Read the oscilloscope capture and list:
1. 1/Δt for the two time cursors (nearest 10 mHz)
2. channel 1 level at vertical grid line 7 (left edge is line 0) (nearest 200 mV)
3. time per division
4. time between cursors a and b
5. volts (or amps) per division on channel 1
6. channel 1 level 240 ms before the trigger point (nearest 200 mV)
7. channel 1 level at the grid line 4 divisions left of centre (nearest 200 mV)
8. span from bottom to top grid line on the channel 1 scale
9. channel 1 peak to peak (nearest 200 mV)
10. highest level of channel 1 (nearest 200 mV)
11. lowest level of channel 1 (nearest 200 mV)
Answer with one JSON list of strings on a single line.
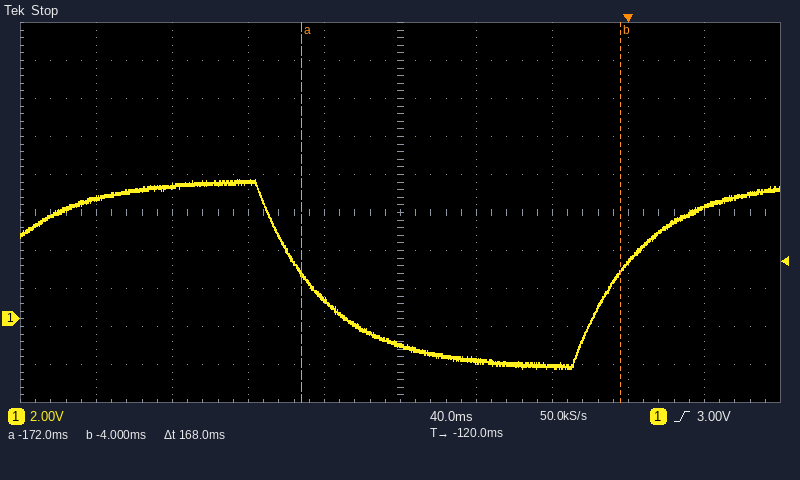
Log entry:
["5.95 Hz", "-2.6 V", "40 ms", "168 ms", "2 V", "7.0 V", "6.4 V", "20 V", "10.0 V", "7.4 V", "-2.6 V"]
